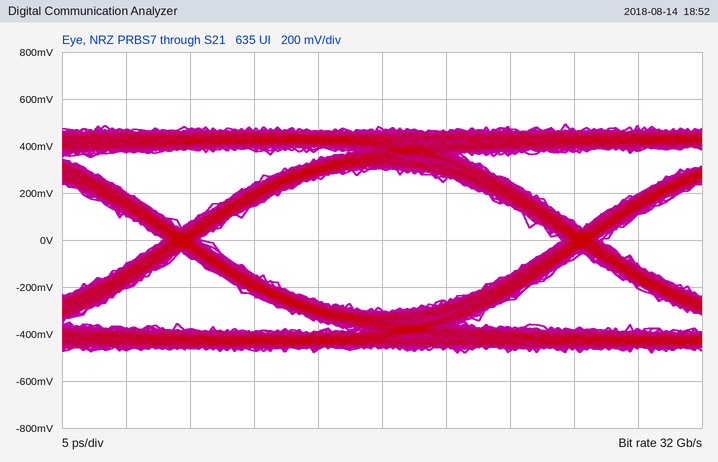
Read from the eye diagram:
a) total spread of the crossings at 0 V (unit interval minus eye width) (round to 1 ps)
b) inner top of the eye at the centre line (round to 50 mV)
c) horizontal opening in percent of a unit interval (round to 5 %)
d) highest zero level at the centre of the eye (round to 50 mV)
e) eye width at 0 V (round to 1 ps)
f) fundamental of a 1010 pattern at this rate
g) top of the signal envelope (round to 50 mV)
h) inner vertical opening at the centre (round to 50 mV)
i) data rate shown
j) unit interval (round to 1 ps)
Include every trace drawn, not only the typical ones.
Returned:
3 ps
300 mV
90 %
-300 mV
28 ps
16 GHz
500 mV
600 mV
32 Gb/s
31 ps
